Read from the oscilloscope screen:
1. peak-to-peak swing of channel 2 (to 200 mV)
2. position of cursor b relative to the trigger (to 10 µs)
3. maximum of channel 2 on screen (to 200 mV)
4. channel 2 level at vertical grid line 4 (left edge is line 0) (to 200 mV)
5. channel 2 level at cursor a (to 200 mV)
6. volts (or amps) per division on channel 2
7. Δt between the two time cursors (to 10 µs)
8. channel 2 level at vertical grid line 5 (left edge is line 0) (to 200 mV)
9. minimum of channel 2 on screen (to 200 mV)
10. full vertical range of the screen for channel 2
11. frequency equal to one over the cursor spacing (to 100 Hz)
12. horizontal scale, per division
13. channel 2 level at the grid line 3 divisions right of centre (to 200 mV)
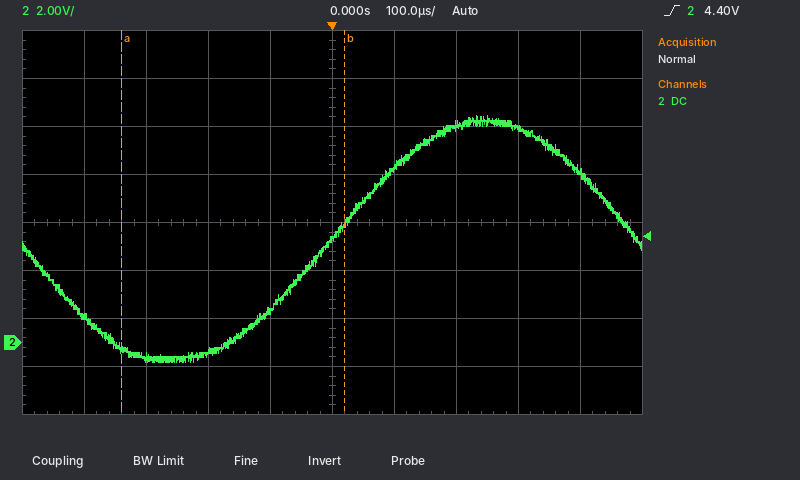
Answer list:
10.2 V
+20 µs
9.4 V
1.4 V
-200 mV
2 V
360 µs
4.4 V
-800 mV
16 V
2.8 kHz
100 µs
9.0 V
